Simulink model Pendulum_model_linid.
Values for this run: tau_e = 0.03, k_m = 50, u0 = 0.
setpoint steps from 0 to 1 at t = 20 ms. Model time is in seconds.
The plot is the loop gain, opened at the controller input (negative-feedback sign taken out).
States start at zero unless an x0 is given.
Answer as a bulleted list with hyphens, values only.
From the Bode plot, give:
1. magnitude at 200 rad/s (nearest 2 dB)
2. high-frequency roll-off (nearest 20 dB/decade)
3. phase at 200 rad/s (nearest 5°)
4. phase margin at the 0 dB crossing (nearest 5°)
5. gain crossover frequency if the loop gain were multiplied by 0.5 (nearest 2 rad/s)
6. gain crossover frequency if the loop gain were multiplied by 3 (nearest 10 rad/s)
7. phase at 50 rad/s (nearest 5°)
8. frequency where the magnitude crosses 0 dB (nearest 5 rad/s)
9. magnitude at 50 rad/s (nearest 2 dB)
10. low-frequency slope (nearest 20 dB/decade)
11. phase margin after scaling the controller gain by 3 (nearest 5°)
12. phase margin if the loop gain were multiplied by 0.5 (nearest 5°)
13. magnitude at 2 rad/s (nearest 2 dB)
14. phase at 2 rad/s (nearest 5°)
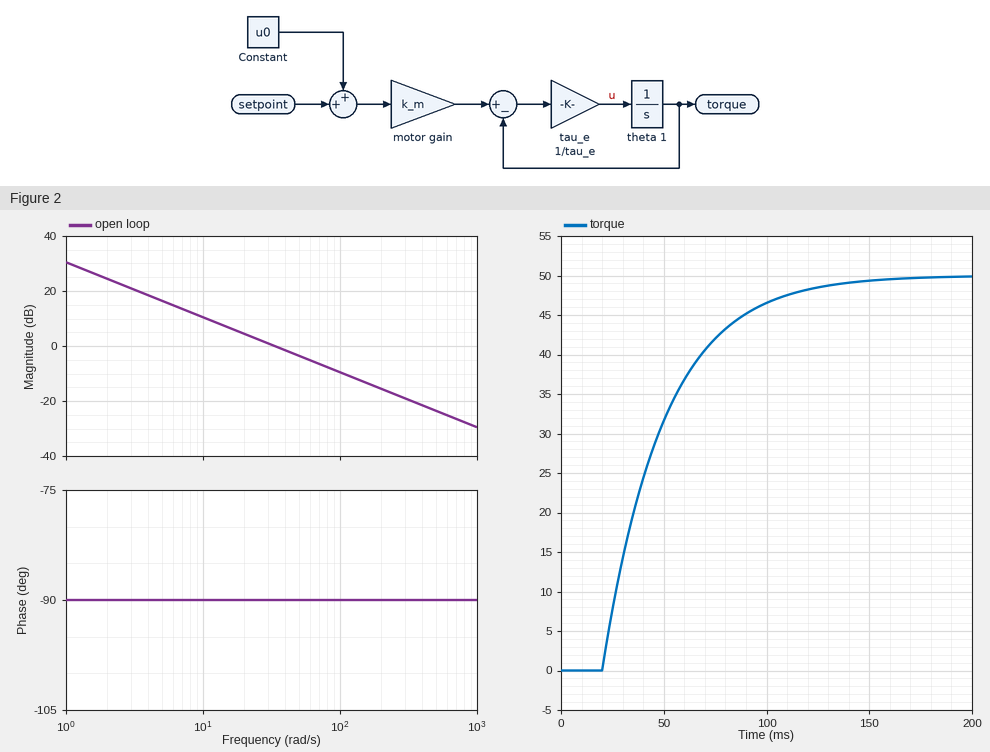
- -16 dB
- -20 dB/decade
- -90°
- 90°
- 16 rad/s
- 100 rad/s
- -90°
- 35 rad/s
- -4 dB
- -20 dB/decade
- 90°
- 90°
- 24 dB
- -90°
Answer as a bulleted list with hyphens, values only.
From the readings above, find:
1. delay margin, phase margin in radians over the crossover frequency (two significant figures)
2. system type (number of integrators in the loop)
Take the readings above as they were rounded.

- 0.045 s
- 1
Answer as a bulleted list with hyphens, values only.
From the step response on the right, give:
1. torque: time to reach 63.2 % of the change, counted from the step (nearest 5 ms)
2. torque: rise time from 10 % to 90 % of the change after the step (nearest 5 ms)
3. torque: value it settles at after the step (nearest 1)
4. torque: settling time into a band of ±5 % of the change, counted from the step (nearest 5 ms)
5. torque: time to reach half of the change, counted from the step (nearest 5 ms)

- 30 ms
- 65 ms
- 50
- 90 ms
- 20 ms
